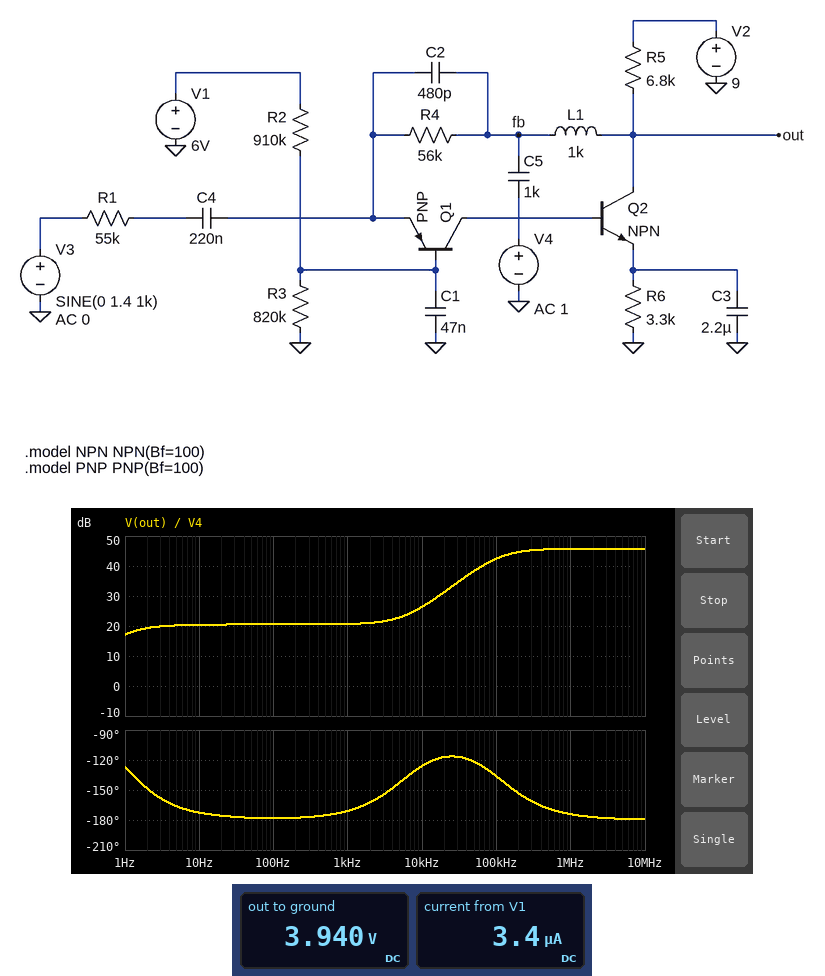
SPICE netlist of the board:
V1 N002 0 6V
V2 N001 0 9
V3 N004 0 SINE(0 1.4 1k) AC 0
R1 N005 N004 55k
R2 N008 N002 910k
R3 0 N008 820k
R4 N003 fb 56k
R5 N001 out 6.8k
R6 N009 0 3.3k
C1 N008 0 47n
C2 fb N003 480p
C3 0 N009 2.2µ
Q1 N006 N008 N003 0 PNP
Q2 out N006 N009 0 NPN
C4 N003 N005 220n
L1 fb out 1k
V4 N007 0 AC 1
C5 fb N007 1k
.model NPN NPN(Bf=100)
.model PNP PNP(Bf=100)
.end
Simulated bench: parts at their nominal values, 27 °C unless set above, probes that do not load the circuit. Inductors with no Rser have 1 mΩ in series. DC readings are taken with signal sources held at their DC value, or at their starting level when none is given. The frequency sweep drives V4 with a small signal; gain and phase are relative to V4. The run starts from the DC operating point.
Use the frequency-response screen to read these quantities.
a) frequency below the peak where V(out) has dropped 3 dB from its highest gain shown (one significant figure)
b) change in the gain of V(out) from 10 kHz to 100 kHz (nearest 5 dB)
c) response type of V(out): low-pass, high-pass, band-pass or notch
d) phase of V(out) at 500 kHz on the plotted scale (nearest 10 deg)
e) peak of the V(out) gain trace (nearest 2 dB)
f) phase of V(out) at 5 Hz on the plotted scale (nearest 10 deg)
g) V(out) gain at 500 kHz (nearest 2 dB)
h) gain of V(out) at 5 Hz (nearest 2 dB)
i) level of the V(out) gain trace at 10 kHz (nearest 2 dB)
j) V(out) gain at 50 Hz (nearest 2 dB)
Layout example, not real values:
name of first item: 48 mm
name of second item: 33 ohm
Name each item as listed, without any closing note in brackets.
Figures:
frequency below the peak where V(out) has dropped 3 dB from its highest gain shown: 100 kHz
change in the gain of V(out) from 10 kHz to 100 kHz: 15 dB
response type of V(out): low-pass, high-pass, band-pass or notch: high-pass
phase of V(out) at 500 kHz on the plotted scale: -170 deg
peak of the V(out) gain trace: 46 dB
phase of V(out) at 5 Hz on the plotted scale: -170 deg
V(out) gain at 500 kHz: 46 dB
gain of V(out) at 5 Hz: 20 dB
level of the V(out) gain trace at 10 kHz: 26 dB
V(out) gain at 50 Hz: 20 dB
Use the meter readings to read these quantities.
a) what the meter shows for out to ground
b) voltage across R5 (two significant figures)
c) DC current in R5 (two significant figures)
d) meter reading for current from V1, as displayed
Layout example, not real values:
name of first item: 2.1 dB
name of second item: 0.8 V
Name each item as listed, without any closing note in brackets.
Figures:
what the meter shows for out to ground: 3.940 V
voltage across R5: 5.1 V
DC current in R5: 740 µA
meter reading for current from V1, as displayed: 3.4 µA
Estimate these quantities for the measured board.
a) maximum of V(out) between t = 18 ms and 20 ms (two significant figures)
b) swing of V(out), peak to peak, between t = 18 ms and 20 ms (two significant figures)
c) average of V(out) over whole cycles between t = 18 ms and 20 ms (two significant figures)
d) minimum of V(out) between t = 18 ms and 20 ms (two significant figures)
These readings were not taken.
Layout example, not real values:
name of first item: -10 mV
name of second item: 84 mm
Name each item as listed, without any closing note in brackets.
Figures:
maximum of V(out) between t = 18 ms and 20 ms: 8.8 V
swing of V(out), peak to peak, between t = 18 ms and 20 ms: 6.9 V
average of V(out) over whole cycles between t = 18 ms and 20 ms: 5.3 V
minimum of V(out) between t = 18 ms and 20 ms: 1.9 V
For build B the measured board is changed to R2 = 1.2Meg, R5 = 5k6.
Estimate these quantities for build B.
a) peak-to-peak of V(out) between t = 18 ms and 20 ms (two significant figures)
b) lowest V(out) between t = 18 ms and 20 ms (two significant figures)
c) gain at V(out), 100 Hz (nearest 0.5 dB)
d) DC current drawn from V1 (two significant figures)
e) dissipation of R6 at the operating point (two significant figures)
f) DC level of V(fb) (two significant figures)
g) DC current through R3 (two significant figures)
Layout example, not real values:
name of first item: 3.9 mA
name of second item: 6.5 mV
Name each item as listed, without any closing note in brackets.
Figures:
peak-to-peak of V(out) between t = 18 ms and 20 ms: 6.4 V
lowest V(out) between t = 18 ms and 20 ms: 2.5 V
gain at V(out), 100 Hz: 9.0 dB
DC current drawn from V1: 2.5 µA
dissipation of R6 at the operating point: 2.4 mW
DC level of V(fb): 4.2 V
DC current through R3: 3.7 µA
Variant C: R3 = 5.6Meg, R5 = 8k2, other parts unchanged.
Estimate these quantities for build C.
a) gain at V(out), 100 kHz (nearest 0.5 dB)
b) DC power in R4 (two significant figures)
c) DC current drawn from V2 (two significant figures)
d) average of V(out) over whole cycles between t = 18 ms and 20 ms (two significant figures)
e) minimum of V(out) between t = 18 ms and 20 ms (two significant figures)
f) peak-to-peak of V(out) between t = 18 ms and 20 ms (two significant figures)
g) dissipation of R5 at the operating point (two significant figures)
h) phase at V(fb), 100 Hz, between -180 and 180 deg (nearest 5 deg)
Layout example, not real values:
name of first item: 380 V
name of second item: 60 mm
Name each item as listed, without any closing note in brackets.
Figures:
gain at V(out), 100 kHz: 40.0 dB
DC power in R4: 740 nW
DC current drawn from V2: 360 µA
average of V(out) over whole cycles between t = 18 ms and 20 ms: 5.7 V
minimum of V(out) between t = 18 ms and 20 ms: 1.5 V
peak-to-peak of V(out) between t = 18 ms and 20 ms: 7.6 V
dissipation of R5 at the operating point: 1.1 mW
phase at V(fb), 100 Hz, between -180 and 180 deg: 0 deg
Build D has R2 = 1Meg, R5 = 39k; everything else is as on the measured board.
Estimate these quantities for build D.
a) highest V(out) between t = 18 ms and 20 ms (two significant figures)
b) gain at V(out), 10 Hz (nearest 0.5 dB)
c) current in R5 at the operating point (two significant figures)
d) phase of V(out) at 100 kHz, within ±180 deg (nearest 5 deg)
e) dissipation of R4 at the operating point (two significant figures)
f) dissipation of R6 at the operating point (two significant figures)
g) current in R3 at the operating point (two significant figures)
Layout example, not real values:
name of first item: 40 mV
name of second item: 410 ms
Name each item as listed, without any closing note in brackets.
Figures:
highest V(out) between t = 18 ms and 20 ms: 8.1 V
gain at V(out), 10 Hz: 32.0 dB
current in R5 at the operating point: 140 µA
phase of V(out) at 100 kHz, within ±180 deg: -165 deg
dissipation of R4 at the operating point: 120 nW
dissipation of R6 at the operating point: 68 µW
current in R3 at the operating point: 3.3 µA
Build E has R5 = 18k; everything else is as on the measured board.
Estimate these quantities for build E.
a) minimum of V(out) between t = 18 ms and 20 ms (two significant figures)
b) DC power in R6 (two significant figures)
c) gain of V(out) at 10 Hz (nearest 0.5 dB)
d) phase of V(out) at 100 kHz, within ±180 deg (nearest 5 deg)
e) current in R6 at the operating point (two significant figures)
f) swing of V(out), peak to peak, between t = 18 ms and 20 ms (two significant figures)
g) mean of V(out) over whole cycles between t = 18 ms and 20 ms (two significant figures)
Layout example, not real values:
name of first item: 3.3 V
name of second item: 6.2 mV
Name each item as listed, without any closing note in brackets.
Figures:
minimum of V(out) between t = 18 ms and 20 ms: 810 mV
DC power in R6: 290 µW
gain of V(out) at 10 Hz: 27.5 dB
phase of V(out) at 100 kHz, within ±180 deg: -155 deg
current in R6 at the operating point: 300 µA
swing of V(out), peak to peak, between t = 18 ms and 20 ms: 7.7 V
mean of V(out) over whole cycles between t = 18 ms and 20 ms: 4.9 V
